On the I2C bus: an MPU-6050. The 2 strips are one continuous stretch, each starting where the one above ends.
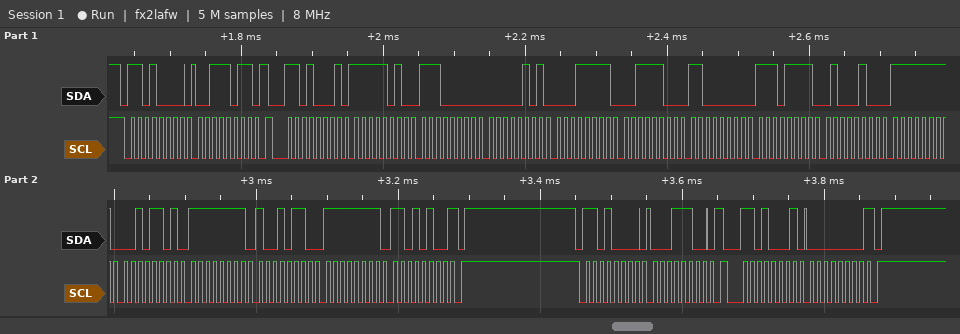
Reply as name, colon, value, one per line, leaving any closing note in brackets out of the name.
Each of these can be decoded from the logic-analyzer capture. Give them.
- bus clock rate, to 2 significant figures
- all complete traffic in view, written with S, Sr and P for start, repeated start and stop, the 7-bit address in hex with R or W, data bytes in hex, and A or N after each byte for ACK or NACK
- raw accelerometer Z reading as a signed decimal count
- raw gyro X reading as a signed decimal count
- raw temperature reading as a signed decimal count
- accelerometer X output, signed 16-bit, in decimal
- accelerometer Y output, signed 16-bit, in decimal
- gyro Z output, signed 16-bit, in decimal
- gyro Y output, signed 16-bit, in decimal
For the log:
bus clock rate, to 2 significant figures: 100 kHz
all complete traffic in view, written with S, Sr and P for start, repeated start and stop, the 7-bit address in hex with R or W, data bytes in hex, and A or N after each byte for ACK or NACK: S 68W A 3B A Sr 68R A FA A E0 A 05 A 1F A 3C A C0 A EF A 44 A FF A 2D A FF A 96 A FF A D4 N P S 68W A 1C A Sr 68R A 00 N P
raw accelerometer Z reading as a signed decimal count: 15552
raw gyro X reading as a signed decimal count: -211
raw temperature reading as a signed decimal count: -4284
accelerometer X output, signed 16-bit, in decimal: -1312
accelerometer Y output, signed 16-bit, in decimal: 1311
gyro Z output, signed 16-bit, in decimal: -44
gyro Y output, signed 16-bit, in decimal: -106
